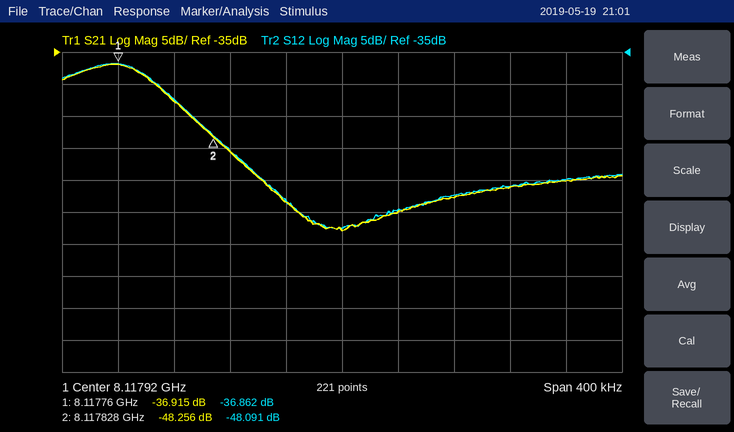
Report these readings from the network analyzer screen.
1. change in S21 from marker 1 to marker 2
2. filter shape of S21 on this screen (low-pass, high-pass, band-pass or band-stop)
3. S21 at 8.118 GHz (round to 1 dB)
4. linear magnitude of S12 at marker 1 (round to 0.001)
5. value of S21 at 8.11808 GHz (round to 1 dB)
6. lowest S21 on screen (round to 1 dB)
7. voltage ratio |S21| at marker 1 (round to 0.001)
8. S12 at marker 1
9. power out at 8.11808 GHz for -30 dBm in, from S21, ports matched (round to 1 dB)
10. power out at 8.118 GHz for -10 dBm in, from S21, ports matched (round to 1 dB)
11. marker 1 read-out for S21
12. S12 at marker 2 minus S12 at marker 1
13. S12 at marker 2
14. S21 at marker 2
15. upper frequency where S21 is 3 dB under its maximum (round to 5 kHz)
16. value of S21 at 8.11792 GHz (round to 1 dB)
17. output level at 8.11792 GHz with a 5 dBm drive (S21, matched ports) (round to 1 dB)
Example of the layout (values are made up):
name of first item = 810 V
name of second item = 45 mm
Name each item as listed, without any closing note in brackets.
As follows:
change in S21 from marker 1 to marker 2 = -11.341 dB
filter shape of S21 on this screen = low-pass
S21 at 8.118 GHz = -58 dB
linear magnitude of S12 at marker 1 = 0.014
value of S21 at 8.11808 GHz = -55 dB
lowest S21 on screen = -63 dB
voltage ratio |S21| at marker 1 = 0.014
S12 at marker 1 = -36.862 dB
power out at 8.11808 GHz for -30 dBm in, from S21, ports matched = -85 dBm
power out at 8.118 GHz for -10 dBm in, from S21, ports matched = -68 dBm
marker 1 read-out for S21 = -36.915 dB
S12 at marker 2 minus S12 at marker 1 = -11.229 dB
S12 at marker 2 = -48.091 dB
S21 at marker 2 = -48.256 dB
upper frequency where S21 is 3 dB under its maximum = 8.117785 GHz
value of S21 at 8.11792 GHz = -63 dB
output level at 8.11792 GHz with a 5 dBm drive (S21, matched ports) = -58 dBm
